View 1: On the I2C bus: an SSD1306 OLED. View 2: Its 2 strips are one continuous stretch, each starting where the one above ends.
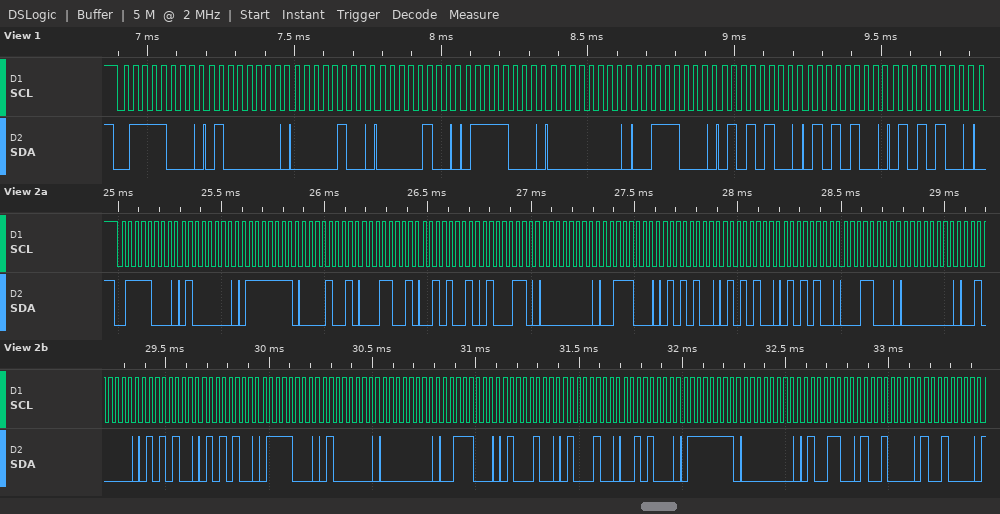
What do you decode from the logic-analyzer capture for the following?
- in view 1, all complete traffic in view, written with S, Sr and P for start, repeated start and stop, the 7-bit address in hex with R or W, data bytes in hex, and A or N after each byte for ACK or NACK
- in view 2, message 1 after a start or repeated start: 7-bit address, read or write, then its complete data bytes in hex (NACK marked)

S 3CW A 40 A 04 A 04 A 78 A 00 A 38 A 54 A 54 A 54 A
0x3C write: 40 7F 09 19 29 46 00 38 54 54 54 18 00 20 54 54 78 40 00 38 44 44 28 7F 00 4C 90 90
